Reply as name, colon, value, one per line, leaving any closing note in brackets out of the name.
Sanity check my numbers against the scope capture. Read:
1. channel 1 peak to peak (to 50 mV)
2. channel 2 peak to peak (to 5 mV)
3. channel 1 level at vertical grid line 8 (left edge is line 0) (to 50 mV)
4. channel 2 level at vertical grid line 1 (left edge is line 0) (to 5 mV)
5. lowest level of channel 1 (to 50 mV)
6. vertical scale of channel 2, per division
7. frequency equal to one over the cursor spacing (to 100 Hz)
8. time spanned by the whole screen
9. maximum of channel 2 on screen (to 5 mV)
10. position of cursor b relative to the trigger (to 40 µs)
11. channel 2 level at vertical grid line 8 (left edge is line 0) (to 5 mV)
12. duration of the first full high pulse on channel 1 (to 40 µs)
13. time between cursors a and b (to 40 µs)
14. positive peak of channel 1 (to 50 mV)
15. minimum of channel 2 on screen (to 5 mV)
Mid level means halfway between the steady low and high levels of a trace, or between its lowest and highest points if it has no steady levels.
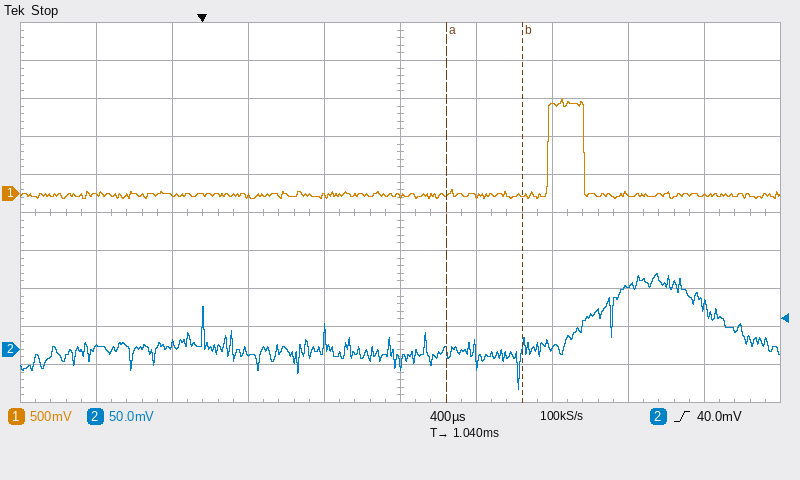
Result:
channel 1 peak to peak: 1.30 V
channel 2 peak to peak: 155 mV
channel 1 level at vertical grid line 8 (left edge is line 0): 0 mV
channel 2 level at vertical grid line 1 (left edge is line 0): 0 mV
lowest level of channel 1: -50 mV
vertical scale of channel 2, per division: 50 mV
frequency equal to one over the cursor spacing: 2.5 kHz
time spanned by the whole screen: 4 ms
maximum of channel 2 on screen: 100 mV
position of cursor b relative to the trigger: +1.68 ms
channel 2 level at vertical grid line 8 (left edge is line 0): 85 mV
duration of the first full high pulse on channel 1: 200 µs
time between cursors a and b: 400 µs
positive peak of channel 1: 1.25 V
minimum of channel 2 on screen: -55 mV
